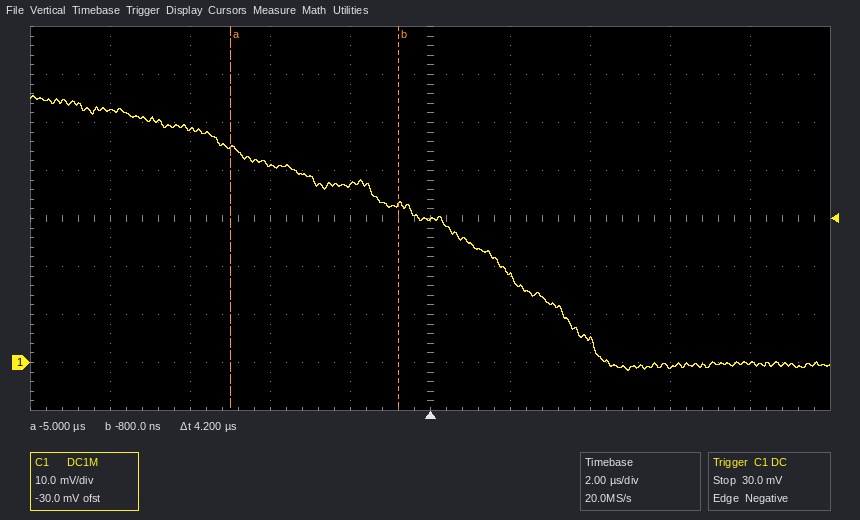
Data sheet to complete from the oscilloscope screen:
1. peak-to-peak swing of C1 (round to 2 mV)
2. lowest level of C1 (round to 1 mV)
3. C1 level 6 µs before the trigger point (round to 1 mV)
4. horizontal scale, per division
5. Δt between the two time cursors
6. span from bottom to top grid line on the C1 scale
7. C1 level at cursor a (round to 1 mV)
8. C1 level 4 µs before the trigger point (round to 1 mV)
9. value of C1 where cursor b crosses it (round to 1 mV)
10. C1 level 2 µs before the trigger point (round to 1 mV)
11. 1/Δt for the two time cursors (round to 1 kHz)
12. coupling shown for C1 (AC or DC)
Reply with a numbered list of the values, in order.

1. 58 mV
2. -2 mV
3. 49 mV
4. 2 µs
5. 4.2 µs
6. 80 mV
7. 45 mV
8. 41 mV
9. 33 mV
10. 37 mV
11. 238 kHz
12. DC
